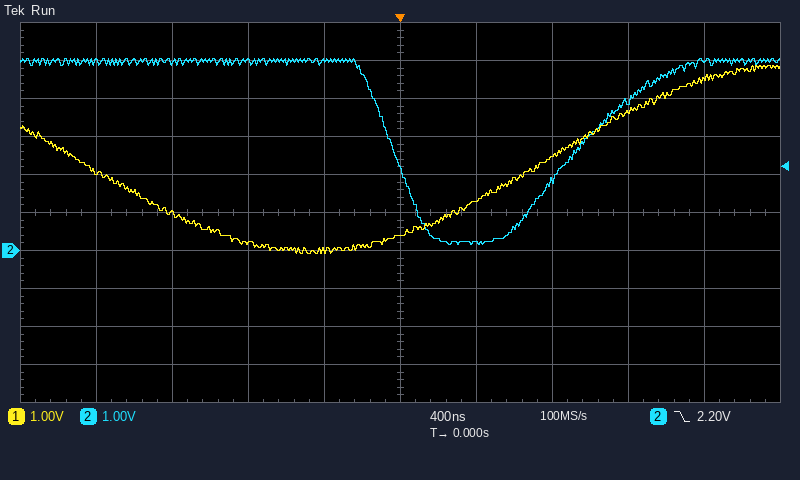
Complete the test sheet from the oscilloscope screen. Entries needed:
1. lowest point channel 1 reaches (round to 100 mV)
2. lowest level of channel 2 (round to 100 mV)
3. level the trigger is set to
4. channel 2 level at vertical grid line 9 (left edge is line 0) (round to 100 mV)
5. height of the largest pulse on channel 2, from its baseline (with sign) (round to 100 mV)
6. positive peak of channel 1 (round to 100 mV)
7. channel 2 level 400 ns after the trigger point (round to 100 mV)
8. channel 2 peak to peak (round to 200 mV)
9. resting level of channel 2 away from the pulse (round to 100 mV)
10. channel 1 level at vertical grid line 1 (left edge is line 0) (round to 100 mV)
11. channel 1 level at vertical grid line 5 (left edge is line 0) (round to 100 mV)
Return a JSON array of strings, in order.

["-100 mV", "200 mV", "2.20 V", "5.0 V", "-4.8 V", "4.9 V", "200 mV", "4.8 V", "5.0 V", "2.1 V", "400 mV"]
